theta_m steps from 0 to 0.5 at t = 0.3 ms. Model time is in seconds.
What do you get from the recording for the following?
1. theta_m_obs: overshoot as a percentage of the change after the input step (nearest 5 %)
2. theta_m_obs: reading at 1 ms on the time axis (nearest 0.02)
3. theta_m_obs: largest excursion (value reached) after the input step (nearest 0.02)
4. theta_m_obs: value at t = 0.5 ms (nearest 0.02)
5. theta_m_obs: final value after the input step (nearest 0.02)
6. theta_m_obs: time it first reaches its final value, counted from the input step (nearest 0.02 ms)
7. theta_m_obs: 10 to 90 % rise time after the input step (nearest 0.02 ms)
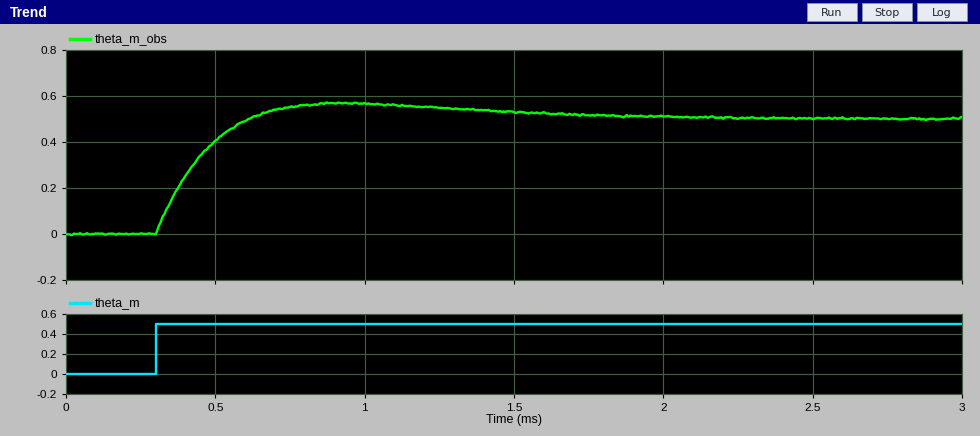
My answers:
15 %
0.56
0.56
0.40
0.50
0.32 ms
0.22 ms
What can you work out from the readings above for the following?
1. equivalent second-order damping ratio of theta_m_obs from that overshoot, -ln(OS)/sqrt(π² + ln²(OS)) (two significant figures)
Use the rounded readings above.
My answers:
0.52
